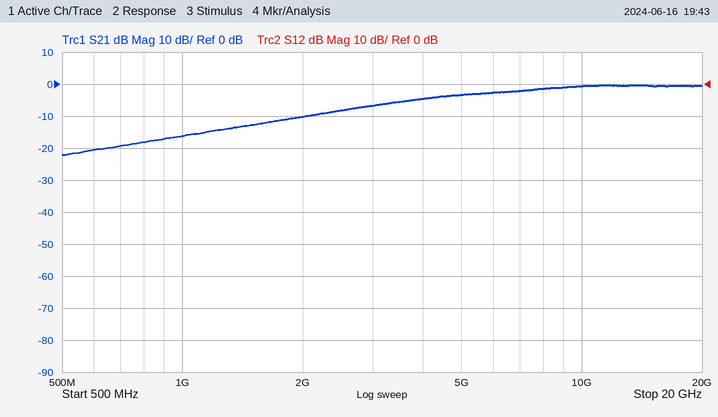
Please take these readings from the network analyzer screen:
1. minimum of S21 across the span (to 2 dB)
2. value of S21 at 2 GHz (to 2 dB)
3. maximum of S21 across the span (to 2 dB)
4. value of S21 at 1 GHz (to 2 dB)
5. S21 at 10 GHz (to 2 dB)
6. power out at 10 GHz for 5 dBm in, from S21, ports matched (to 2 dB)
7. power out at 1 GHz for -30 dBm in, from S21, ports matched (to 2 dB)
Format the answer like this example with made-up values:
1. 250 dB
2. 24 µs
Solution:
1. -22 dB
2. -10 dB
3. 0 dB
4. -16 dB
5. 0 dB
6. 4 dBm
7. -46 dBm
